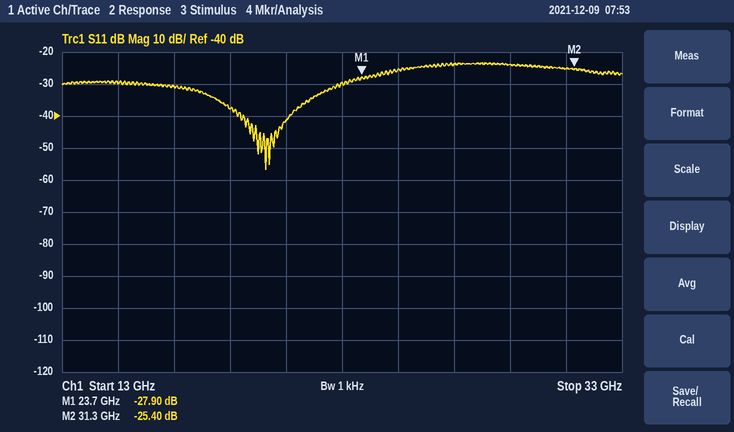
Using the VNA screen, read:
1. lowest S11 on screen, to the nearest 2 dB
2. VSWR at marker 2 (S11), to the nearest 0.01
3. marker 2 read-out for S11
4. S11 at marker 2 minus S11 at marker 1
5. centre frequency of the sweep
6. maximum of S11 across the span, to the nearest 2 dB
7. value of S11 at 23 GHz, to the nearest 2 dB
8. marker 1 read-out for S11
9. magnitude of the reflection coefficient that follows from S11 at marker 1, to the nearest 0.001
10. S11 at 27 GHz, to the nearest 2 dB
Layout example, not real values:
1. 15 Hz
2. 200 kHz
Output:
1. -56 dB
2. 1.11
3. -25.40 dB
4. 2.50 dB
5. 23 GHz
6. -24 dB
7. -30 dB
8. -27.90 dB
9. 0.040
10. -24 dB
